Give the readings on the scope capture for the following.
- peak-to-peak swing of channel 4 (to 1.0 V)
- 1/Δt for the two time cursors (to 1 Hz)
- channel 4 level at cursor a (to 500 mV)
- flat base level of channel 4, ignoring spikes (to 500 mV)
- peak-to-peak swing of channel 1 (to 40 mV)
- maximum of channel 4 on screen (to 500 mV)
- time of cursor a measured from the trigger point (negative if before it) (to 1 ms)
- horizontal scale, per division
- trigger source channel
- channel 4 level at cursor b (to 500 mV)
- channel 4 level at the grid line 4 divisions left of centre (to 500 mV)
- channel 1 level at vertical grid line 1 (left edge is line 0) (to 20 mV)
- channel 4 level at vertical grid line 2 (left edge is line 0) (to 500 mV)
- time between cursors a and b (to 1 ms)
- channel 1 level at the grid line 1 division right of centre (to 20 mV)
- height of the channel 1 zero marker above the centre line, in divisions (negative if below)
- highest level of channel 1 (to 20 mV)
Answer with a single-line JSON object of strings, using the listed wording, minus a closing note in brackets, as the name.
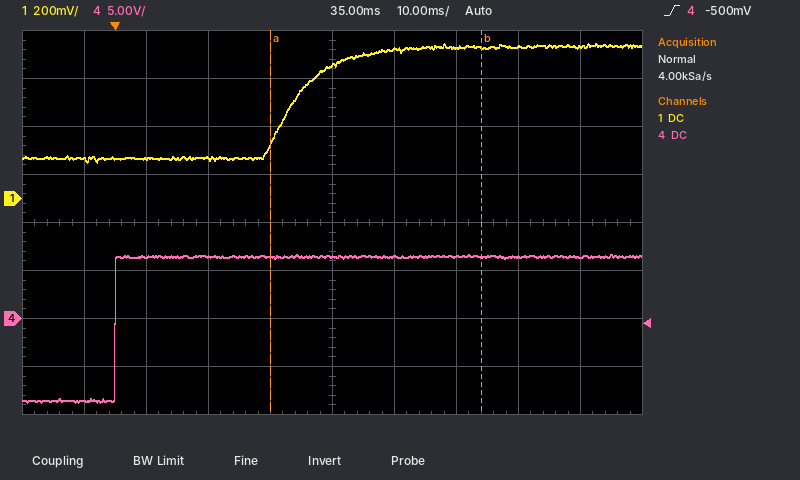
{"peak-to-peak swing of channel 4": "15.0 V", "1/Δt for the two time cursors": "29 Hz", "channel 4 level at cursor a": "6.5 V", "flat base level of channel 4, ignoring spikes": "-8.5 V", "peak-to-peak swing of channel 1": "480 mV", "maximum of channel 4 on screen": "6.5 V", "time of cursor a measured from the trigger point (negative if before it)": "+25 ms", "horizontal scale, per division": "10 ms", "trigger source channel": "channel 4", "channel 4 level at cursor b": "6.5 V", "channel 4 level at the grid line 4 divisions left of centre": "-8.5 V", "channel 1 level at vertical grid line 1 (left edge is line 0)": "160 mV", "channel 4 level at vertical grid line 2 (left edge is line 0)": "6.5 V", "time between cursors a and b": "34 ms", "channel 1 level at the grid line 1 division right of centre": "620 mV", "height of the channel 1 zero marker above the centre line, in divisions": "+0.5 div", "highest level of channel 1": "640 mV"}
